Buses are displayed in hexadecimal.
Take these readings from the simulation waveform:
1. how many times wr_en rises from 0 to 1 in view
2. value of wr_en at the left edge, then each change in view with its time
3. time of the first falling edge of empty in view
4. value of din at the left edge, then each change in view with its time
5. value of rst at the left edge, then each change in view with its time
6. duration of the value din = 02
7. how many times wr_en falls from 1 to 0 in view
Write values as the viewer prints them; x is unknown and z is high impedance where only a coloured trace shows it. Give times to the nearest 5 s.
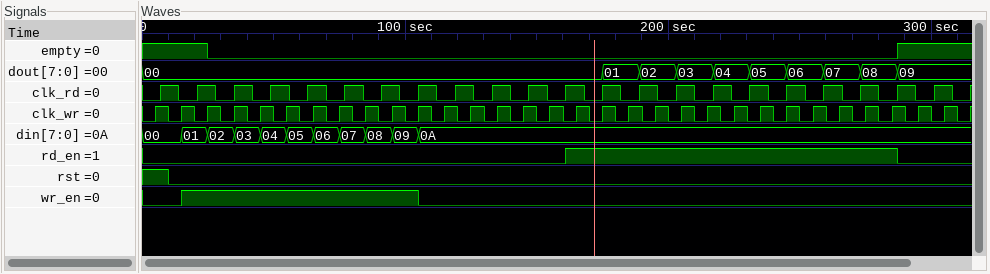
1
0, 1 at 15 s, 0 at 105 s
25 s
00, 01 at 15 s, 02 at 25 s, 03 at 35 s, 04 at 45 s, 05 at 55 s, 06 at 65 s, 07 at 75 s, 08 at 85 s, 09 at 95 s, 0A at 105 s
1, 0 at 10 s
10 s
1
